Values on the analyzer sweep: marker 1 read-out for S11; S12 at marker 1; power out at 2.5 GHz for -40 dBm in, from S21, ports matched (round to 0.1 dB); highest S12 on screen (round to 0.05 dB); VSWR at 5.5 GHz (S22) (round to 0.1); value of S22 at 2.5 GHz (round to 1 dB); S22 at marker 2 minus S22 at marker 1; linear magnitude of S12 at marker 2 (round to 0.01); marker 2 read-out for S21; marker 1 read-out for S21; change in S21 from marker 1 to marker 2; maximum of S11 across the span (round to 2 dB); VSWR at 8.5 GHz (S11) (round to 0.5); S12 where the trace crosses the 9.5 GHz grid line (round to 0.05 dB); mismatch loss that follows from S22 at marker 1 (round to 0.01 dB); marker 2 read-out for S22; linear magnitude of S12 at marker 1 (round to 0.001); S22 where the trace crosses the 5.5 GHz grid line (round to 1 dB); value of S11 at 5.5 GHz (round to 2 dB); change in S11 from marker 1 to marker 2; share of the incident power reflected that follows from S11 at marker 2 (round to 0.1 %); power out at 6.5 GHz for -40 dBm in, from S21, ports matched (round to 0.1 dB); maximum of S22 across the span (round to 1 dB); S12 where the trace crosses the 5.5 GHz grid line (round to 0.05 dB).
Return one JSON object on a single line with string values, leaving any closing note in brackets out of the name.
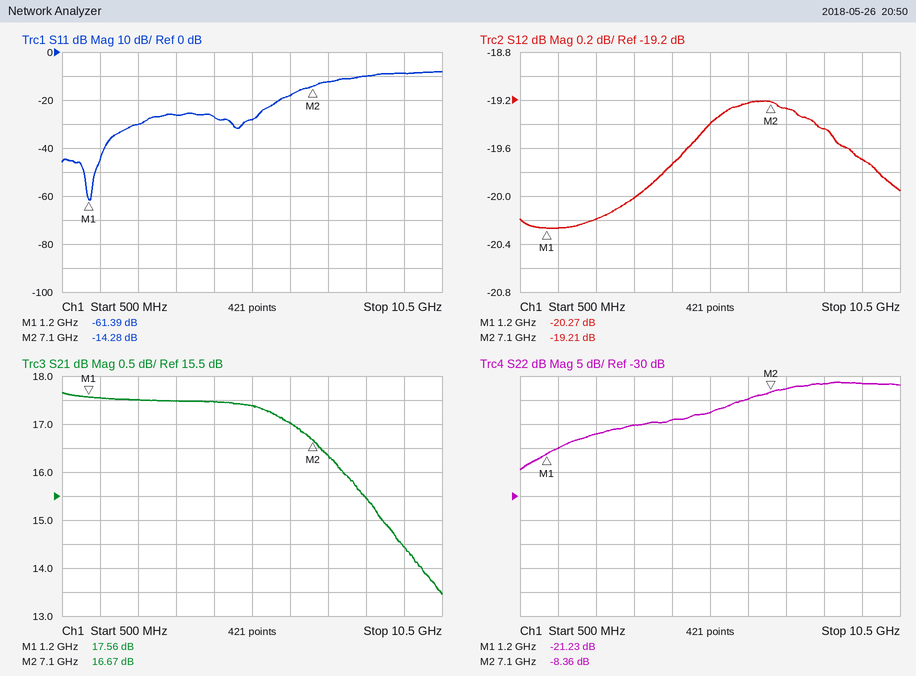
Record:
{"marker 1 read-out for S11": "-61.39 dB", "S12 at marker 1": "-20.27 dB", "power out at 2.5 GHz for -40 dBm in, from S21, ports matched": "-22.5 dBm", "highest S12 on screen": "-19.20 dB", "VSWR at 5.5 GHz (S22)": "1.6", "value of S22 at 2.5 GHz": "-17 dB", "S22 at marker 2 minus S22 at marker 1": "12.87 dB", "linear magnitude of S12 at marker 2": "0.11", "marker 2 read-out for S21": "16.67 dB", "marker 1 read-out for S21": "17.56 dB", "change in S21 from marker 1 to marker 2": "-0.89 dB", "maximum of S11 across the span": "-8 dB", "VSWR at 8.5 GHz (S11)": "2.0", "S12 where the trace crosses the 9.5 GHz grid line": "-19.70 dB", "mismatch loss that follows from S22 at marker 1": "0.03 dB", "marker 2 read-out for S22": "-8.36 dB", "linear magnitude of S12 at marker 1": "0.097", "S22 where the trace crosses the 5.5 GHz grid line": "-13 dB", "value of S11 at 5.5 GHz": "-28 dB", "change in S11 from marker 1 to marker 2": "47.11 dB", "share of the incident power reflected that follows from S11 at marker 2": "3.7 %", "power out at 6.5 GHz for -40 dBm in, from S21, ports matched": "-23.0 dBm", "maximum of S22 across the span": "-6 dB", "S12 where the trace crosses the 5.5 GHz grid line": "-19.40 dB"}
